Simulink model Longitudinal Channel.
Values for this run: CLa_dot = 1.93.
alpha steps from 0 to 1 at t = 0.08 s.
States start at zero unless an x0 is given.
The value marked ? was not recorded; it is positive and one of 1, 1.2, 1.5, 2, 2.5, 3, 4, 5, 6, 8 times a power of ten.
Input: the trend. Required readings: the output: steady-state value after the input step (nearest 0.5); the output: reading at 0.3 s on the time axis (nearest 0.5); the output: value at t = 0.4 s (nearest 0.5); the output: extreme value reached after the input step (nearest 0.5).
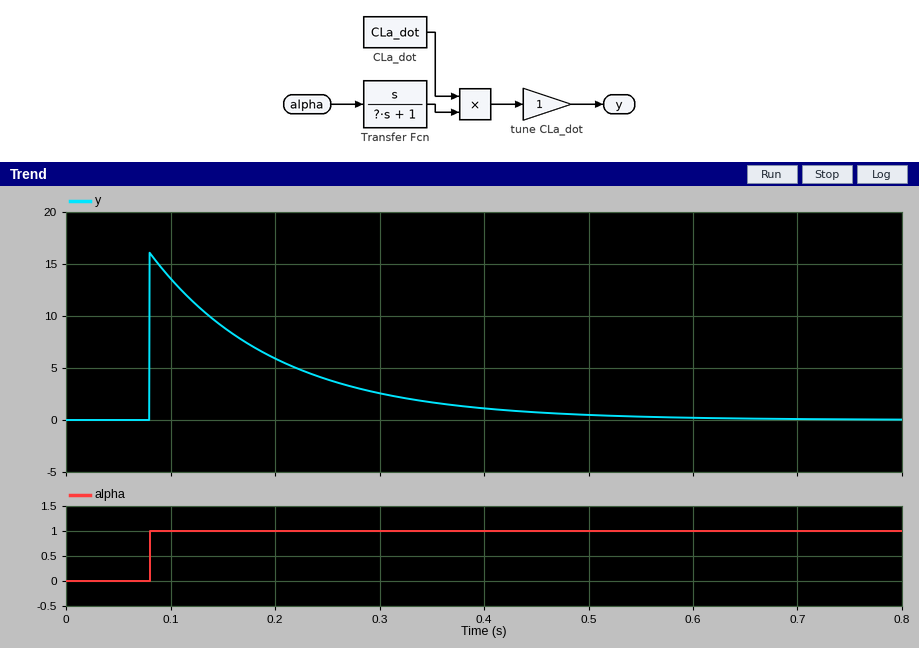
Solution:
0.0
2.5
1.0
16.0
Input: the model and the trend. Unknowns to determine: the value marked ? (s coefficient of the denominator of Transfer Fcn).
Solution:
0.12
